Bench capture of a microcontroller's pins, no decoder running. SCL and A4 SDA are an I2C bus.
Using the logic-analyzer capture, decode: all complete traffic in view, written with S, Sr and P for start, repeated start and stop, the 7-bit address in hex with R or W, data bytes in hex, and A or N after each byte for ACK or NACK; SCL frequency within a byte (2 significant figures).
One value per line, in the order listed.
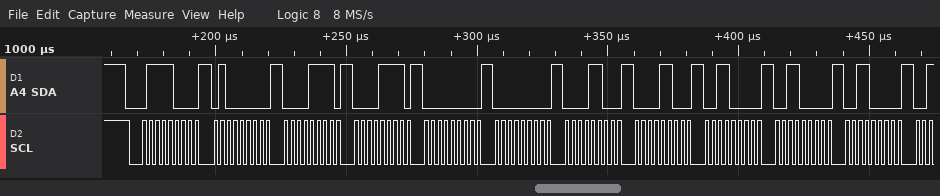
S 3CW A 40 A 0F A 0F A 00 A 00 A 0C A 0C A 30 A 30 A 30 A
400 kHz
